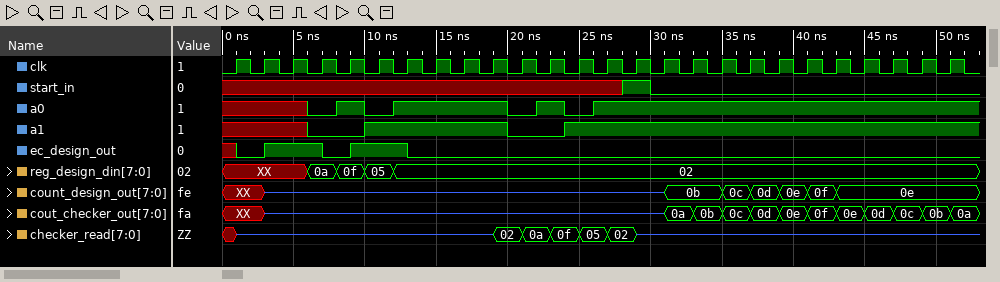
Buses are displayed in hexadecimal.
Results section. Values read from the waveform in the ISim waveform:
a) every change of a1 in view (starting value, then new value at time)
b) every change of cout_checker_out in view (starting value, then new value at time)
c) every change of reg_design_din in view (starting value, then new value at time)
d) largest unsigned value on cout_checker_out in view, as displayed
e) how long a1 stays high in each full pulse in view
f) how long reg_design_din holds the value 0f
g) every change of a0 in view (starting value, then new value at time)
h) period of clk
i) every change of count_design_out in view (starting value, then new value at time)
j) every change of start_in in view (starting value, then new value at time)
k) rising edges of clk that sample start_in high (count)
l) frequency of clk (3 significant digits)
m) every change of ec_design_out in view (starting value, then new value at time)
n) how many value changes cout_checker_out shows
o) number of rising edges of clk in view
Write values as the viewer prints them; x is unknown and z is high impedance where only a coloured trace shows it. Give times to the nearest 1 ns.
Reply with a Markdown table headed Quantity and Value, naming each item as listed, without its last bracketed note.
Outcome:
| Quantity | Value |
|---|---|
| every change of a1 in view | x, 0 at 6 ns, 1 at 10 ns, 0 at 20 ns, 1 at 24 ns |
| every change of cout_checker_out in view | XX, z at 3 ns, 0a at 31 ns, 0b at 33 ns, 0c at 35 ns, 0d at 37 ns, 0e at 39 ns, 0f at 41 ns, 0e at 43 ns, 0d at 45 ns, 0c at 47 ns, 0b at 49 ns, 0a at 51 ns |
| every change of reg_design_din in view | XX, 0a at 6 ns, 0f at 8 ns, 05 at 10 ns, 02 at 12 ns |
| largest unsigned value on cout_checker_out in view, as displayed | 0f |
| how long a1 stays high in each full pulse in view | 10 ns |
| how long reg_design_din holds the value 0f | 2 ns |
| every change of a0 in view | x, 0 at 6 ns, 1 at 8 ns, 0 at 10 ns, 1 at 12 ns, 0 at 20 ns, 1 at 22 ns, 0 at 24 ns, 1 at 26 ns |
| period of clk | 2 ns |
| every change of count_design_out in view | XX, z at 3 ns, 0b at 31 ns, 0c at 35 ns, 0d at 37 ns, 0e at 39 ns, 0f at 41 ns, 0e at 43 ns |
| every change of start_in in view | x, 1 at 28 ns, 0 at 30 ns |
| rising edges of clk that sample start_in high | 1 |
| frequency of clk | 500 MHz |
| every change of ec_design_out in view | x, 0 at 1 ns, 1 at 3 ns, 0 at 7 ns, 1 at 9 ns, 0 at 13 ns |
| how many value changes cout_checker_out shows | 12 |
| number of rising edges of clk in view | 26 |
